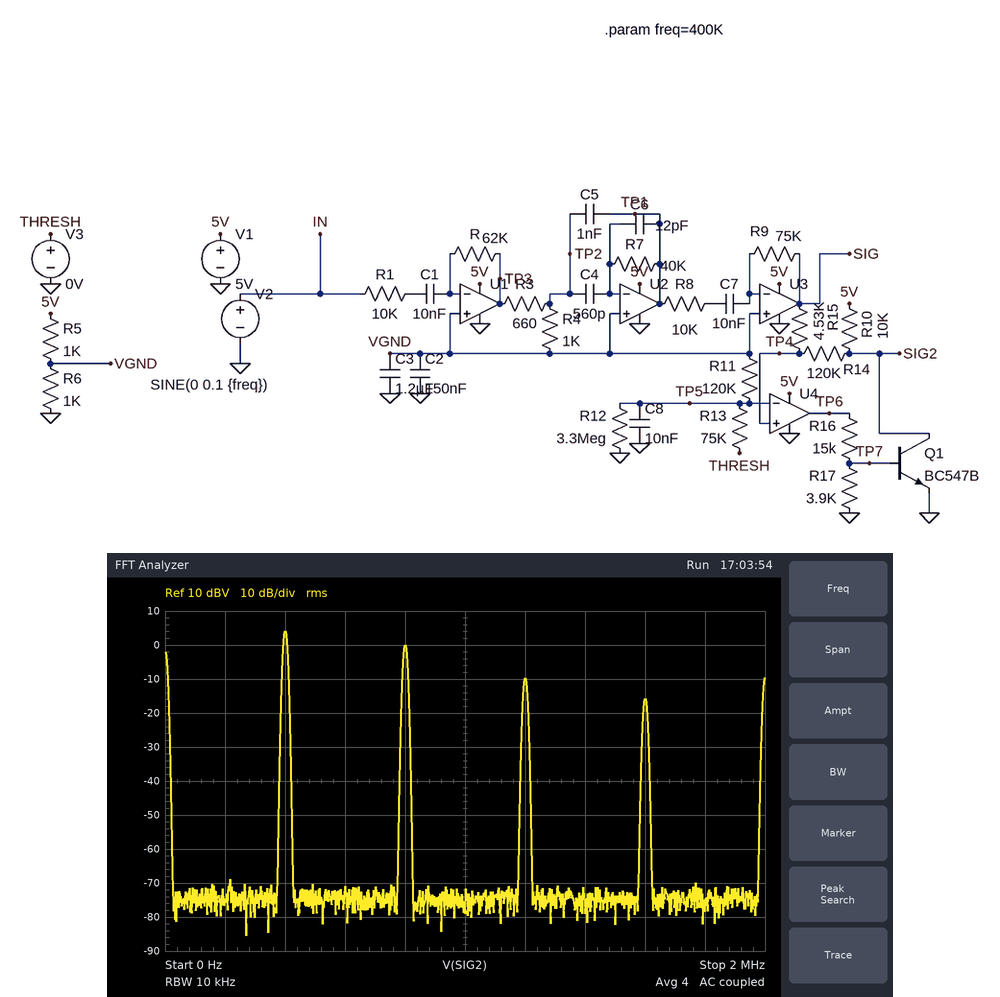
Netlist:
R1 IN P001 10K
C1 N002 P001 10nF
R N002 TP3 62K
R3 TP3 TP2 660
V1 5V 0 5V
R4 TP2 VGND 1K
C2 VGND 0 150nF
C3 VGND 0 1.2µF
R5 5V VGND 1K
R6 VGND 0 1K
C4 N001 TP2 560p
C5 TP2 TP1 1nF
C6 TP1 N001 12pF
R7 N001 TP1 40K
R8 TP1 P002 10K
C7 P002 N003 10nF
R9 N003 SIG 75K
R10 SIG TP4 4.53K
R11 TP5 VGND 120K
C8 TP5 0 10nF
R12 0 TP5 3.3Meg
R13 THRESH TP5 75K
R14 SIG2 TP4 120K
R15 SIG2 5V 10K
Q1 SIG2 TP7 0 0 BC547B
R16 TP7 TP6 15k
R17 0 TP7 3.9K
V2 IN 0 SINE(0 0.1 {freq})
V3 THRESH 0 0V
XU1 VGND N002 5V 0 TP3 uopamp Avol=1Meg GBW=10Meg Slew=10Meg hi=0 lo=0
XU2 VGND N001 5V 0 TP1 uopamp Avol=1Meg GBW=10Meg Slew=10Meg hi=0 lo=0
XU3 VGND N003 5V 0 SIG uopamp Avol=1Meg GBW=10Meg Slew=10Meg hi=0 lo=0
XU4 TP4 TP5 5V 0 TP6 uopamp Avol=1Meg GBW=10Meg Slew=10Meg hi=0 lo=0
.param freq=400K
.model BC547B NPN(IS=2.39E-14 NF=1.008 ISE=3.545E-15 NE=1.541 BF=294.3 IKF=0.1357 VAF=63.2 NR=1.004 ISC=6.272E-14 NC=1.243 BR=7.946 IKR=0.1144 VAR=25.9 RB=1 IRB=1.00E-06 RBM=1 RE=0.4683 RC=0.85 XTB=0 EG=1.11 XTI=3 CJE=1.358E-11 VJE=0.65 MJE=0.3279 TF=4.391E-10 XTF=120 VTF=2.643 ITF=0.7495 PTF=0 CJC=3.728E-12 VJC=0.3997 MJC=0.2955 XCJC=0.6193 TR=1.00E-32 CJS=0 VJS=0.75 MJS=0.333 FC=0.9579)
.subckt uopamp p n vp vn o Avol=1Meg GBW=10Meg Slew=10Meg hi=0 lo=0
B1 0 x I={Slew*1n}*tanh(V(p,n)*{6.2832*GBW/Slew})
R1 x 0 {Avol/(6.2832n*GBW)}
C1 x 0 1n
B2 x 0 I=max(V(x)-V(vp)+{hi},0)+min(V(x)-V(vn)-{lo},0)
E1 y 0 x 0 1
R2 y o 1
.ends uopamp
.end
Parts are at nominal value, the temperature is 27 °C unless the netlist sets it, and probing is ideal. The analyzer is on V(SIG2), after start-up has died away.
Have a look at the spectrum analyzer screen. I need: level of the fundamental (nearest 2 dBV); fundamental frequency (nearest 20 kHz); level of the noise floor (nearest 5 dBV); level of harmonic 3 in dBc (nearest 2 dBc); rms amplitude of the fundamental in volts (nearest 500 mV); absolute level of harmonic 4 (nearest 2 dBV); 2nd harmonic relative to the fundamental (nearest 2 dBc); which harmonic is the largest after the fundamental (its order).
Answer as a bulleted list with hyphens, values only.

- 4 dBV
- 400 kHz
- -75 dBV
- -14 dBc
- 1.5 V
- -16 dBV
- -4 dBc
- 2
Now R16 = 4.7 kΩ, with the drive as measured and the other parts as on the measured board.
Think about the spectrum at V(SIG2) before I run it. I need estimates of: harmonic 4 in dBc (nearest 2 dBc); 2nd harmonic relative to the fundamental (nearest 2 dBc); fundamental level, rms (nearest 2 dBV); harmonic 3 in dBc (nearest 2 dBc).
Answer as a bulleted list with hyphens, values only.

- -6 dBc
- -2 dBc
- 0 dBV
- -4 dBc
